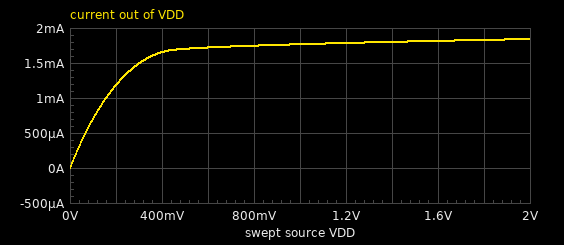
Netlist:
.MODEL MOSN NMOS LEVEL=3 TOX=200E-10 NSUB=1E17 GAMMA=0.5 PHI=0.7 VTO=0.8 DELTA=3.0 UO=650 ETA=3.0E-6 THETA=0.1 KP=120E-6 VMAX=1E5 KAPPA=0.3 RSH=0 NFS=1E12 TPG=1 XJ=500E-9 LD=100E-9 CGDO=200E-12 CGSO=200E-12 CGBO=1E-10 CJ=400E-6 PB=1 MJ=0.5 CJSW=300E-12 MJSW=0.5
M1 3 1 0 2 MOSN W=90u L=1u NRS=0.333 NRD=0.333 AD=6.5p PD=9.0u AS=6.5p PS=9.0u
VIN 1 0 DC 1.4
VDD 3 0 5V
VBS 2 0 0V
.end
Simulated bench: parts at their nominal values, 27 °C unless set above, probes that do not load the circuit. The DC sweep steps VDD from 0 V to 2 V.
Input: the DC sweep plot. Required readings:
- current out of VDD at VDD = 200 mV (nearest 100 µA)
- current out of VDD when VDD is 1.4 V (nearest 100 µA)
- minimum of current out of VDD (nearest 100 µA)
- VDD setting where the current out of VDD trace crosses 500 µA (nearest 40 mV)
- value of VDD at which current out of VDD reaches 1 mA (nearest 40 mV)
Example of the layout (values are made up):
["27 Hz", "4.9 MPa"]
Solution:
["1.2 mA", "1.8 mA", "0 A", "80 mV", "160 mV"]
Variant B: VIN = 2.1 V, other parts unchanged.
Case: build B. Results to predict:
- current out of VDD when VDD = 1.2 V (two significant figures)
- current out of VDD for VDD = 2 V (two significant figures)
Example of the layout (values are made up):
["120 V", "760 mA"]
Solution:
["5.6 mA", "5.8 mA"]
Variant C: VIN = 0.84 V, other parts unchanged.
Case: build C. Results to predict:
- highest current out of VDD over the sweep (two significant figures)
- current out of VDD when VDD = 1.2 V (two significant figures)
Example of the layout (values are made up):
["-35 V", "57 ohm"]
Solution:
["51 µA", "50 µA"]
